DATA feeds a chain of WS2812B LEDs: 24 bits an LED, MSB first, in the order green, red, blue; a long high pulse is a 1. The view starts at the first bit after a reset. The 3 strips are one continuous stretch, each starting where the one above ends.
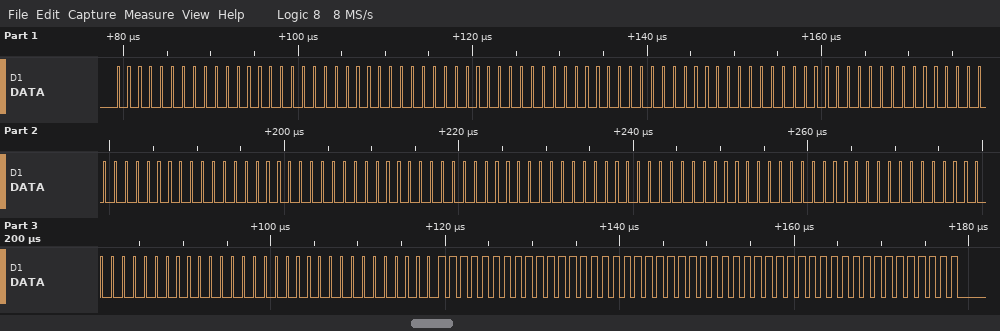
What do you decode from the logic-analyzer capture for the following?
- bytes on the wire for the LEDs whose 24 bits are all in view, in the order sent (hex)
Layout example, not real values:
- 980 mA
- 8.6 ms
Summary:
- 00 00 00 00 00 00 00 00 00 00 00 00 00 00 00 00 00 00 00 00 00 00 00 00 FF FF FF FF FF FF
